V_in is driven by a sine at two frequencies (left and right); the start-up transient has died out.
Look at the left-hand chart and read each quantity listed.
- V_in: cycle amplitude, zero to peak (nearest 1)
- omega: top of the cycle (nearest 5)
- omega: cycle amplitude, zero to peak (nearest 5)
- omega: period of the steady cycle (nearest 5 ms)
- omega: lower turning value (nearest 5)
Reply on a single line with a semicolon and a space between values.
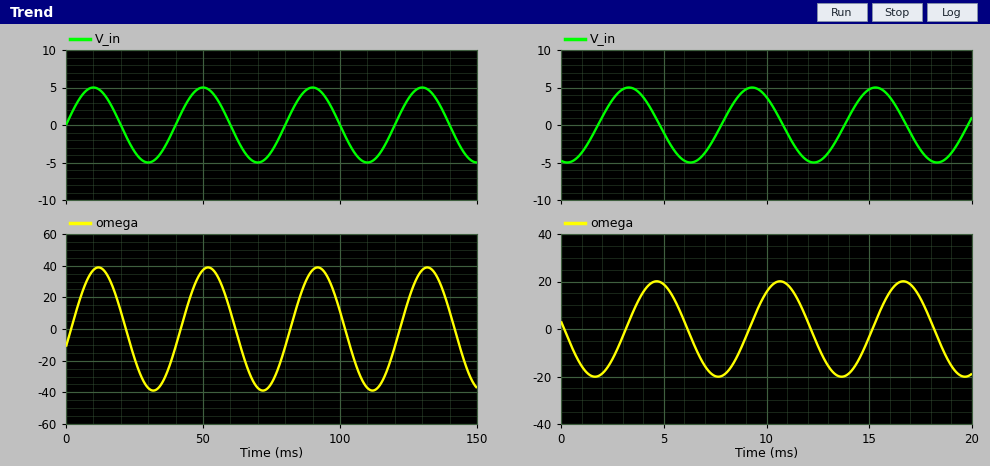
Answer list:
5; 40; 40; 40 ms; -40
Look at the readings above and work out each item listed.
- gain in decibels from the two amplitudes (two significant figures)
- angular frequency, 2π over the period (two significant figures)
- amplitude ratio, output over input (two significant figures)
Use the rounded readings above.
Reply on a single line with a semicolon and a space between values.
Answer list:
18 dB; 0.16 rad/ms; 8.0
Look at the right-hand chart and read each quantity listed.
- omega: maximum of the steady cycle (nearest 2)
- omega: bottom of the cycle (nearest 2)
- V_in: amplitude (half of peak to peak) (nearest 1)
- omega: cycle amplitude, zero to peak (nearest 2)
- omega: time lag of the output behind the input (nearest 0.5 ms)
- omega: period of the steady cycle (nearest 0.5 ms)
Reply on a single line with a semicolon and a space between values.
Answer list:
20; -20; 5; 20; 1.5 ms; 6.0 ms
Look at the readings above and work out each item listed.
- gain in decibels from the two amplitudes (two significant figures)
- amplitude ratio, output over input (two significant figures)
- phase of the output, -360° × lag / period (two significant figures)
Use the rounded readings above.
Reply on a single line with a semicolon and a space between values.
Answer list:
12 dB; 4.0; -90°
